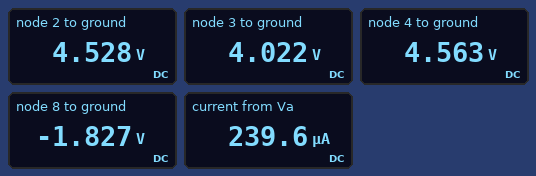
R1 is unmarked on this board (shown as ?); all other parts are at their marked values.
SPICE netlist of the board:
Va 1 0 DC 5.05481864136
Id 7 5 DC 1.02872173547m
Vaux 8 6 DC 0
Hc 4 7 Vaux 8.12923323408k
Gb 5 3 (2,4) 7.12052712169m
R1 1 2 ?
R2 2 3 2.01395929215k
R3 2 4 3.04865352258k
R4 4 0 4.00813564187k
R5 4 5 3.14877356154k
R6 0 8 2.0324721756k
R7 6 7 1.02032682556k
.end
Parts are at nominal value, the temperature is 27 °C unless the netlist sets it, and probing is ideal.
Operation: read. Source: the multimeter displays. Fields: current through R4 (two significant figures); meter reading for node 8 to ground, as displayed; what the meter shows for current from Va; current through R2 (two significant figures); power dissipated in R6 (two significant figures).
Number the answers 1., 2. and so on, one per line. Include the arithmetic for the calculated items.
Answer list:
1. (4.563 V) / 4.008 kΩ = 1.1 mA
2. -1.827 V
3. 239.6 µA
4. (4.528 V - 4.022 V) / 2.014 kΩ = 250 µA
5. (0 V - (-1.827 V))^2 / 2.032 kΩ = 1.6 mW
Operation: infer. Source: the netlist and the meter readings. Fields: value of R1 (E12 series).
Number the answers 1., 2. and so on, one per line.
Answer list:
1. 2.2 kΩ
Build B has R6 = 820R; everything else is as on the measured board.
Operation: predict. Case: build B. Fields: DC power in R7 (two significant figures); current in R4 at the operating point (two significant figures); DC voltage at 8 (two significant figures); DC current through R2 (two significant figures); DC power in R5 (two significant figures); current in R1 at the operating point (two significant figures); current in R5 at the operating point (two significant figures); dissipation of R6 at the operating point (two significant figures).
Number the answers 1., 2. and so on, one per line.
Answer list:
1. 470 µW
2. 1.1 mA
3. -560 mV
4. 400 µA
5. 6.5 mW
6. 390 µA
7. 1.4 mA
8. 380 µW
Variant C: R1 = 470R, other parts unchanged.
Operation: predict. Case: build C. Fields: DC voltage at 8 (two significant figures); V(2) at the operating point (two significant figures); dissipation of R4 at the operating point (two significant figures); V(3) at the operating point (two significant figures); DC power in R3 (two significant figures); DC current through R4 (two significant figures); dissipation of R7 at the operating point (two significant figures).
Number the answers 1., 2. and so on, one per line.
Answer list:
1. -2.0 V
2. 4.9 V
3. 6.2 mW
4. 4.4 V
5. 480 nW
6. 1.2 mA
7. 980 µW
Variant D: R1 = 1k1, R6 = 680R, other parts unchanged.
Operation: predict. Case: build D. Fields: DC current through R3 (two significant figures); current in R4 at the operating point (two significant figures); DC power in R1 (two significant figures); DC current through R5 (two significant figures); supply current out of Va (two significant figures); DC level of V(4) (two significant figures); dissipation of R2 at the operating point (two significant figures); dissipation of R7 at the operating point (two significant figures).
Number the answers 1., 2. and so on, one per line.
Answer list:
1. 21 µA
2. 1.2 mA
3. 210 µW
4. 1.5 mA
5. 440 µA
6. 4.6 V
7. 420 µW
8. 530 µW
